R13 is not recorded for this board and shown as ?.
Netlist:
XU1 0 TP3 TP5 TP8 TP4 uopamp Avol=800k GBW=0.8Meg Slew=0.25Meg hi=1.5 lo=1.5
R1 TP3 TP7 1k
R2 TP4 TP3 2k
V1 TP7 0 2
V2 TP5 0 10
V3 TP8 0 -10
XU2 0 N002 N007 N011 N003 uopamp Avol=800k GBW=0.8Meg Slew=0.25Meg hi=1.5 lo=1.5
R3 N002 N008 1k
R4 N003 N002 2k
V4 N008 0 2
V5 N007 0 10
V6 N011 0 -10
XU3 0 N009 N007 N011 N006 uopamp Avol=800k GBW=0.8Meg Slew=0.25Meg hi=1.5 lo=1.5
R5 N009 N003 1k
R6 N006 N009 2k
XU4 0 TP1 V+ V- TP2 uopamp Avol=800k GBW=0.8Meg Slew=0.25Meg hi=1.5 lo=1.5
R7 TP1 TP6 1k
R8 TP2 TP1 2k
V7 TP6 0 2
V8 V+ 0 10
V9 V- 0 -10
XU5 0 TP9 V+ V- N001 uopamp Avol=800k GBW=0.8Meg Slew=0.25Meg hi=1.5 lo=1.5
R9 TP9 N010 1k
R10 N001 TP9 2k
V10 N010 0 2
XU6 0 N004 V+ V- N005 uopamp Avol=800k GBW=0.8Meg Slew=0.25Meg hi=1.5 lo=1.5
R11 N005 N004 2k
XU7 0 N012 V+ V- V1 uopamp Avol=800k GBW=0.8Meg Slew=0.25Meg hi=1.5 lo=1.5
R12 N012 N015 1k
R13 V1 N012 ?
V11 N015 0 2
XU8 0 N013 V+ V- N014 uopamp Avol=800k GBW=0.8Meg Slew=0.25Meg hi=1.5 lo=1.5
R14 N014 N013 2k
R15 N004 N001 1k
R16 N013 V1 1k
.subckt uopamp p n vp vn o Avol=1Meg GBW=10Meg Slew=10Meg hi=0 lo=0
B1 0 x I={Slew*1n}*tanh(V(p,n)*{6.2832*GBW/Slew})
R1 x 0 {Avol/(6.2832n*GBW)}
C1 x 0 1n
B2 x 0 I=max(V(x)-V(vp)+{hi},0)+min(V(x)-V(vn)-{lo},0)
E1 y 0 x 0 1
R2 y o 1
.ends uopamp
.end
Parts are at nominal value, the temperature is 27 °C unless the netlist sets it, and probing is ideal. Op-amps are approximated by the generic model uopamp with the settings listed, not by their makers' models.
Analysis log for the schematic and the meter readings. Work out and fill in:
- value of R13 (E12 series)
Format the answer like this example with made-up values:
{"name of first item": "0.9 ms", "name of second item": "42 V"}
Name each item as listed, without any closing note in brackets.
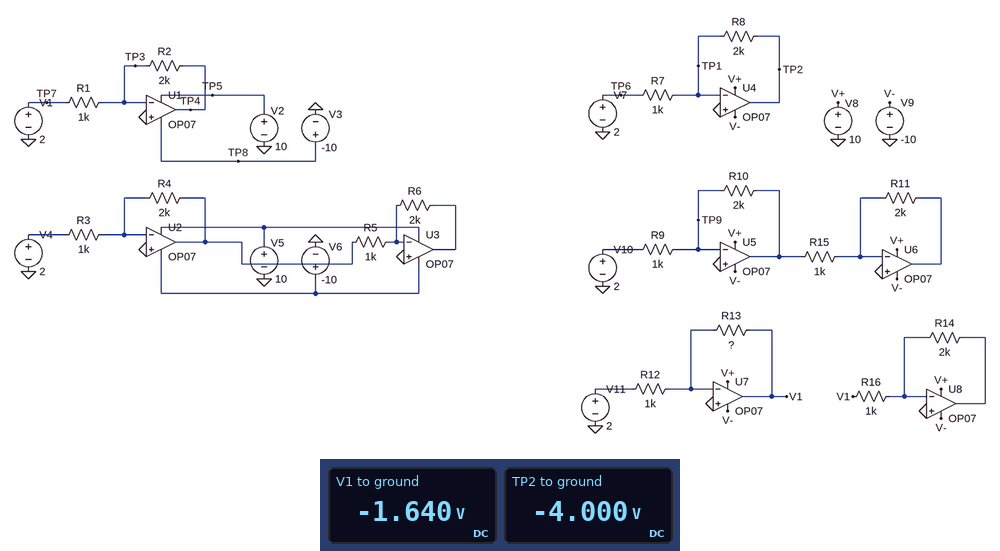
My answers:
{"value of R13": "820 Ω"}
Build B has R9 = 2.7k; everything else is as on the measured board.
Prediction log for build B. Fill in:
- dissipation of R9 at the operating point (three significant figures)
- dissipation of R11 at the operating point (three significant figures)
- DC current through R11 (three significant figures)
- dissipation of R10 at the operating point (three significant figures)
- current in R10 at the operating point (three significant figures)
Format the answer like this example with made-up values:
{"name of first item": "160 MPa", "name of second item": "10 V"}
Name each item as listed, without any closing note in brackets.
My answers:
{"dissipation of R9 at the operating point": "1.48 mW", "dissipation of R11 at the operating point": "4.39 mW", "DC current through R11": "1.48 mA", "dissipation of R10 at the operating point": "1.10 mW", "current in R10 at the operating point": "741 µA"}
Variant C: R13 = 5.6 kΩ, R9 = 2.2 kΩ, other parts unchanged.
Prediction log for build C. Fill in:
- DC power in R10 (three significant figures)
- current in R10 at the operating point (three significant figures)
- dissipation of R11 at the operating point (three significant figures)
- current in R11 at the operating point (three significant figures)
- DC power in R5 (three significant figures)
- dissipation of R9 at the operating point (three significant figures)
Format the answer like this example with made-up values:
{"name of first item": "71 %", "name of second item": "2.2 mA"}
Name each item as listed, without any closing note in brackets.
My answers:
{"DC power in R10": "1.65 mW", "current in R10 at the operating point": "909 µA", "dissipation of R11 at the operating point": "6.61 mW", "current in R11 at the operating point": "1.82 mA", "DC power in R5": "16.0 mW", "dissipation of R9 at the operating point": "1.82 mW"}
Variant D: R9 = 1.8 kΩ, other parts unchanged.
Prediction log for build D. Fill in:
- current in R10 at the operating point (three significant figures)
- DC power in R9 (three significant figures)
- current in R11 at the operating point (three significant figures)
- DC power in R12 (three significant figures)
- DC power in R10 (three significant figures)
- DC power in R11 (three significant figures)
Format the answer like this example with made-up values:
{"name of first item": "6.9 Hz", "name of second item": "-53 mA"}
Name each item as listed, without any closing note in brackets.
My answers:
{"current in R10 at the operating point": "1.11 mA", "DC power in R9": "2.22 mW", "current in R11 at the operating point": "2.22 mA", "DC power in R12": "4.00 mW", "DC power in R10": "2.47 mW", "DC power in R11": "9.88 mW"}
